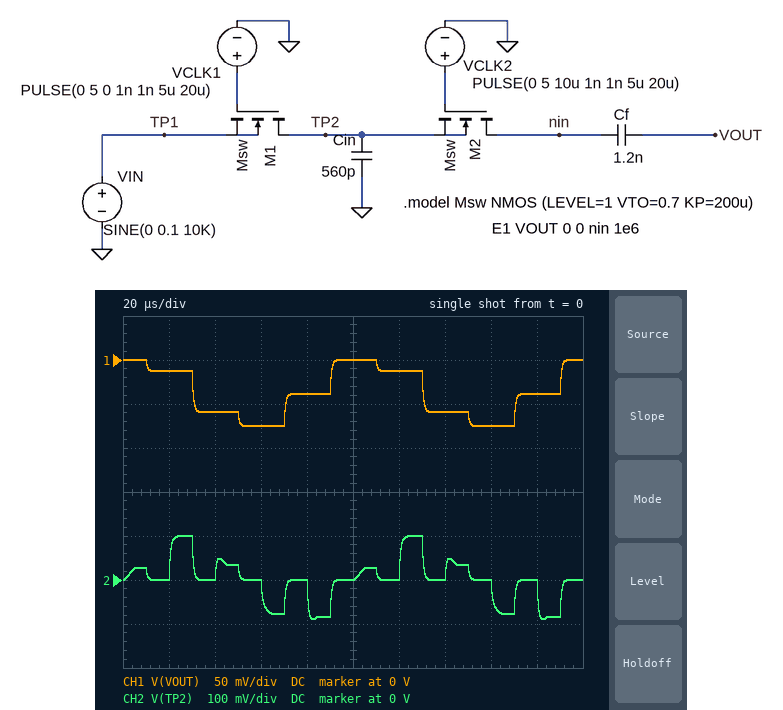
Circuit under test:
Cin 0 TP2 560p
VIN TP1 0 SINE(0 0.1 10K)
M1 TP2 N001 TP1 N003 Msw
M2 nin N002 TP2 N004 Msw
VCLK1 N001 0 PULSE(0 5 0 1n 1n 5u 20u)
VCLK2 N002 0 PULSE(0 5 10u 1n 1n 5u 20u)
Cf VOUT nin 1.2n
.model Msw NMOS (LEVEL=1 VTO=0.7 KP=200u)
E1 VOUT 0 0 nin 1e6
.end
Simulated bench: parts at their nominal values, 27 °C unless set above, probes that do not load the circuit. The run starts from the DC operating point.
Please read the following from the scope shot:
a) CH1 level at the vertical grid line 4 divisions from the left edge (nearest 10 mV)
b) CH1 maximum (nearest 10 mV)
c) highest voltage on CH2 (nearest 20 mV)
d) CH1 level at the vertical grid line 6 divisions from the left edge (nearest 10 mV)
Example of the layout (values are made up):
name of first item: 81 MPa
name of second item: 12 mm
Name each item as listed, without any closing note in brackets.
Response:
CH1 level at the vertical grid line 4 divisions from the left edge: -40 mV
CH1 maximum: 0 V
highest voltage on CH2: 100 mV
CH1 level at the vertical grid line 6 divisions from the left edge: -10 mV
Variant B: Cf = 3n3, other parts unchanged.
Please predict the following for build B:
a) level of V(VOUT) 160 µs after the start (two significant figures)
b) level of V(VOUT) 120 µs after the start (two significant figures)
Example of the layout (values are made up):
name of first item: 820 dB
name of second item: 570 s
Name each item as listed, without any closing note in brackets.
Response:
level of V(VOUT) 160 µs after the start: -27 mV
level of V(VOUT) 120 µs after the start: -4.6 mV
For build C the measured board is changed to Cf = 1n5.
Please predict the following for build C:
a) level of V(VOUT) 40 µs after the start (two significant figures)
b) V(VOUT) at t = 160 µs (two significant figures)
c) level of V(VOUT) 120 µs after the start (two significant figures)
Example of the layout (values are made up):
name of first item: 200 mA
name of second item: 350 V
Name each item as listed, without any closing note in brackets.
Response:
level of V(VOUT) 40 µs after the start: -47 mV
V(VOUT) at t = 160 µs: -60 mV
level of V(VOUT) 120 µs after the start: -10 mV
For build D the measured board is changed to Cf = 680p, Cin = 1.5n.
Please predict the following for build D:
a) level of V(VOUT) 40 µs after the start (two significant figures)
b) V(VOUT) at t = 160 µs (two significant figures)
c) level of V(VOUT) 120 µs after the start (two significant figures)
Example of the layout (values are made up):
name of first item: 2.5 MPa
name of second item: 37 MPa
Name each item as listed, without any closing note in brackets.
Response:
level of V(VOUT) 40 µs after the start: -240 mV
V(VOUT) at t = 160 µs: -310 mV
level of V(VOUT) 120 µs after the start: -41 mV
